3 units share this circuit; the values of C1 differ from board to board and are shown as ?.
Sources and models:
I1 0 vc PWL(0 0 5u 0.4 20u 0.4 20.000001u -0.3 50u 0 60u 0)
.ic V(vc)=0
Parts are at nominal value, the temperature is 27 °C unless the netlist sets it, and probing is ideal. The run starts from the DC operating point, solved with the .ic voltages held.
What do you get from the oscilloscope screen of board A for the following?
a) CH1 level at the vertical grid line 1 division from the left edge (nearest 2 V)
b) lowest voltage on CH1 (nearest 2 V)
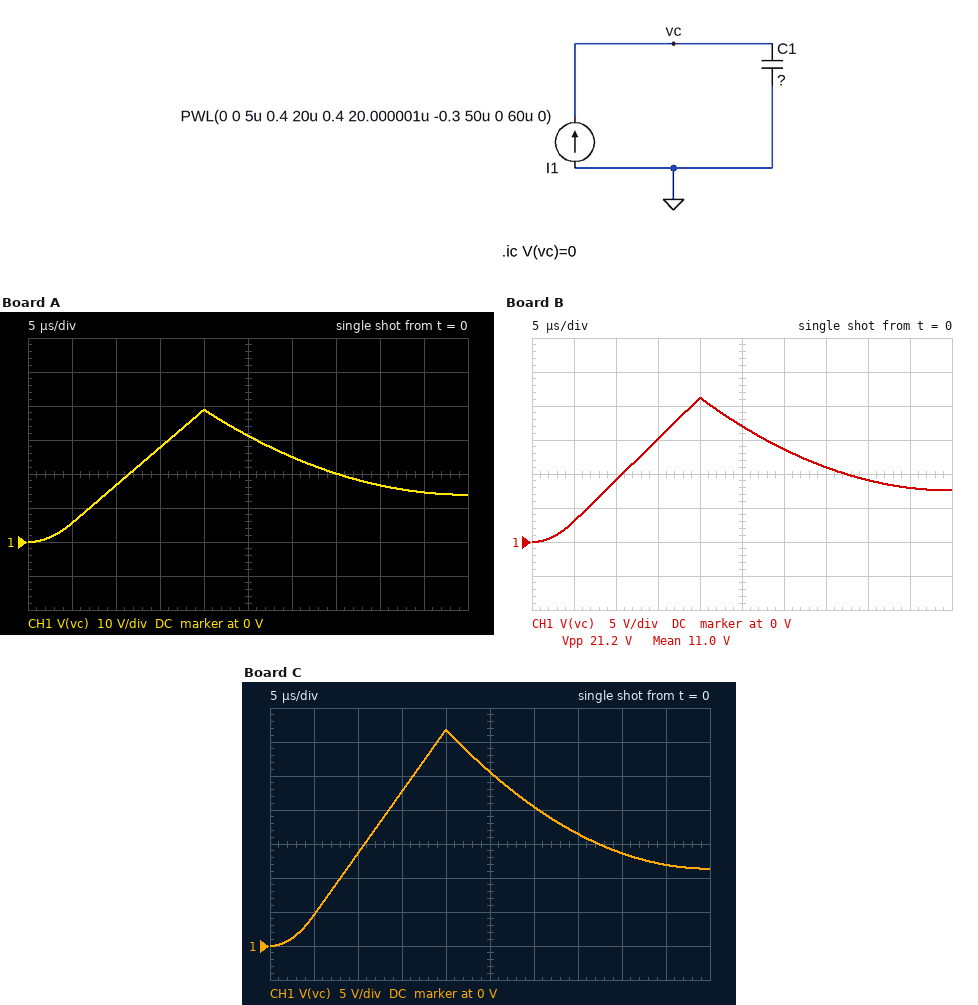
6 V
0 V
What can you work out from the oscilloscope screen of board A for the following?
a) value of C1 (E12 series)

180 nF
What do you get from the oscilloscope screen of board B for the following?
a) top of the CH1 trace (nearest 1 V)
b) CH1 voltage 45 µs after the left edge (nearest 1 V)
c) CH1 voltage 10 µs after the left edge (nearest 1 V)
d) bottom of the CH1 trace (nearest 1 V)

21 V
8 V
9 V
0 V
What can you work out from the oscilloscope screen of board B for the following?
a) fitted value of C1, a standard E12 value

330 nF
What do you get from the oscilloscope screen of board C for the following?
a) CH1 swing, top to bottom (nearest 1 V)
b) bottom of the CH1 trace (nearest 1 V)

32 V
0 V
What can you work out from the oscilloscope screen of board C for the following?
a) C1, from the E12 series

220 nF
